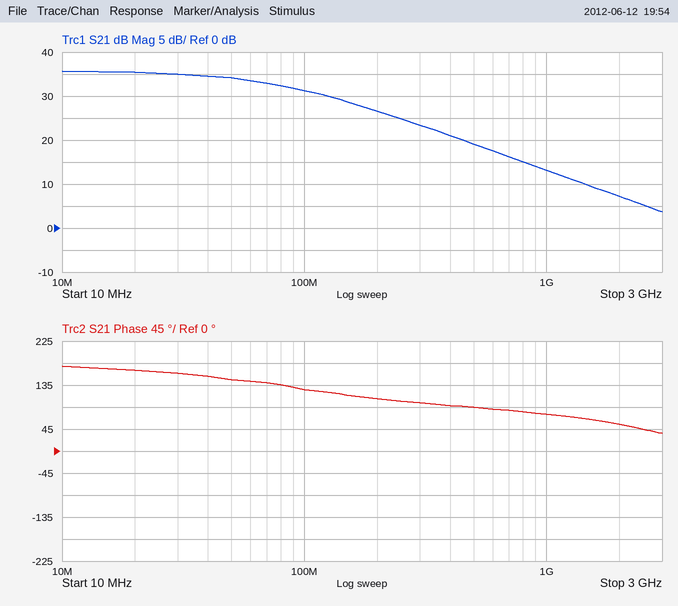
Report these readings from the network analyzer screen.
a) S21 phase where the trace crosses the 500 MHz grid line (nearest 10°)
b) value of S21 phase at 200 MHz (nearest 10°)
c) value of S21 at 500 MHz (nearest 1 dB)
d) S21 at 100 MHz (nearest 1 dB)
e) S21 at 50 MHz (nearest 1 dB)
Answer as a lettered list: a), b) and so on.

a) 90°
b) 110°
c) 19 dB
d) 31 dB
e) 34 dB
